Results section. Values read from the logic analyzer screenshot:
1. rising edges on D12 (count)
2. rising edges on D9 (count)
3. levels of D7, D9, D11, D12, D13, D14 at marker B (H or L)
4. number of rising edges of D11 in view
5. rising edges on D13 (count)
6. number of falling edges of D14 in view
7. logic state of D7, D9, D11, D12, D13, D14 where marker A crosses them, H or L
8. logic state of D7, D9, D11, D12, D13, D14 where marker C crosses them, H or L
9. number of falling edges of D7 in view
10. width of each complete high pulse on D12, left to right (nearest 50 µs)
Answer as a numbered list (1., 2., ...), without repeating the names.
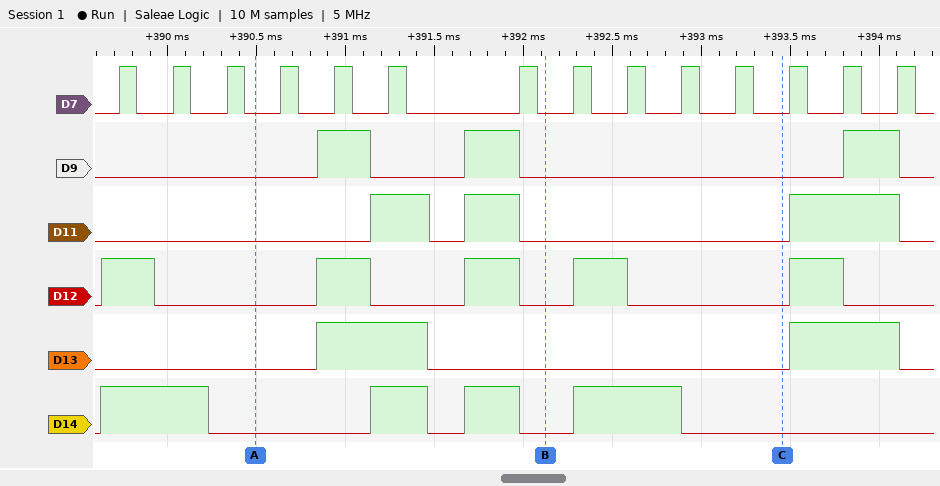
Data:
1. 5
2. 3
3. D7=L, D9=L, D11=L, D12=L, D13=L, D14=L
4. 3
5. 2
6. 4
7. D7=L, D9=L, D11=L, D12=L, D13=L, D14=L
8. D7=L, D9=L, D11=L, D12=L, D13=L, D14=L
9. 14
10. 300 µs, 300 µs, 300 µs, 300 µs, 300 µs
